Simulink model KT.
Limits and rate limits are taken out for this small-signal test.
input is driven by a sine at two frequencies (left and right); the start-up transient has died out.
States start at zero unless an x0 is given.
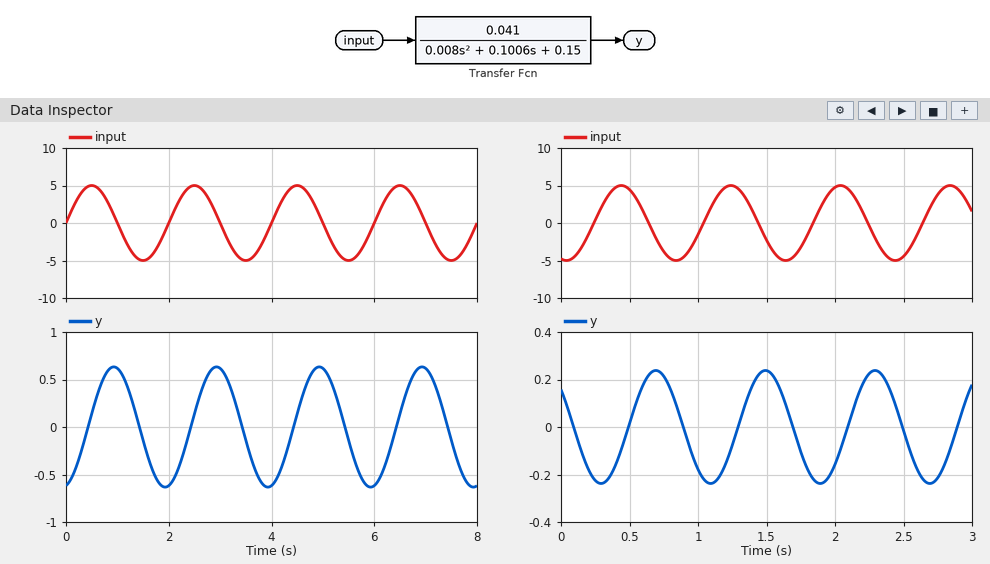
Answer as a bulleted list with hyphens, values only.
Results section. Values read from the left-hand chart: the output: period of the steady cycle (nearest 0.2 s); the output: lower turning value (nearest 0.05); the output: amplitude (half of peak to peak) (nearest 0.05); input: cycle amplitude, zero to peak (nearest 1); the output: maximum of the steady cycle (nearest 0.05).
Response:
- 2.0 s
- -0.65
- 0.65
- 5
- 0.65
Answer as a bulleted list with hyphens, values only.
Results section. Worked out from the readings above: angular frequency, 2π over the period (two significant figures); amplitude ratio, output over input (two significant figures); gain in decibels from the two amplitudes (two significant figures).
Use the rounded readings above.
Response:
- 3.1 rad/s
- 0.13
- -18 dB
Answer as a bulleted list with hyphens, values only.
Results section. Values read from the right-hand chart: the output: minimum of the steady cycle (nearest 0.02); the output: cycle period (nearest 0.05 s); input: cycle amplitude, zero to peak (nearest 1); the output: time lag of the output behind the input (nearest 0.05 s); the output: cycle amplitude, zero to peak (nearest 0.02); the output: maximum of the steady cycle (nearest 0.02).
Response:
- -0.24
- 0.80 s
- 5
- 0.25 s
- 0.24
- 0.24
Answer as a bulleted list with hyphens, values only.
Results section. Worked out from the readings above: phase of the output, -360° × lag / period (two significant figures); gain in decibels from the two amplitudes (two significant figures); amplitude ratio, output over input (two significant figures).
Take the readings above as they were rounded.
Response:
- -110°
- -26 dB
- 0.048
